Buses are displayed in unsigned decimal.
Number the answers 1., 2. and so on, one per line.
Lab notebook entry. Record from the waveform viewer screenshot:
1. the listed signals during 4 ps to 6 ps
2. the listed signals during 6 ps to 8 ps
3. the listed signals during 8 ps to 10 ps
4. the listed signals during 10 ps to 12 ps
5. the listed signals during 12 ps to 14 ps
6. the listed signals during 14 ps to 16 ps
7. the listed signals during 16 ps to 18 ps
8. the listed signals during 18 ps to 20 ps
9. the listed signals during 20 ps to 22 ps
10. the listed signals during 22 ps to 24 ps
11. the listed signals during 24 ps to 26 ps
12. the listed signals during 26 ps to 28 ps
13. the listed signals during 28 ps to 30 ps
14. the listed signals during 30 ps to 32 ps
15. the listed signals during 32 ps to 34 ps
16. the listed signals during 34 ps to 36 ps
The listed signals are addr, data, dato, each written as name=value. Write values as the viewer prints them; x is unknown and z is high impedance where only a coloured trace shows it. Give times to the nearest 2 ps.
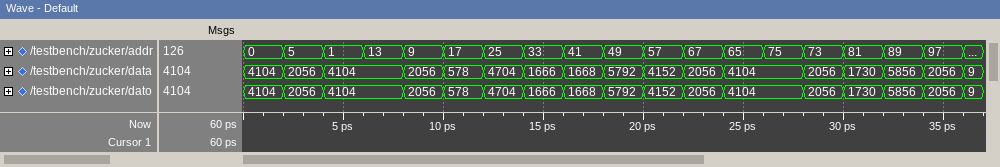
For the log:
1. addr=1, data=4104, dato=4104
2. addr=13, data=4104, dato=4104
3. addr=9, data=2056, dato=2056
4. addr=17, data=578, dato=578
5. addr=25, data=4704, dato=4704
6. addr=33, data=1666, dato=1666
7. addr=41, data=1668, dato=1668
8. addr=49, data=5792, dato=5792
9. addr=57, data=4152, dato=4152
10. addr=67, data=2056, dato=2056
11. addr=65, data=4104, dato=4104
12. addr=75, data=4104, dato=4104
13. addr=73, data=2056, dato=2056
14. addr=81, data=1730, dato=1730
15. addr=89, data=5856, dato=5856
16. addr=97, data=2056, dato=2056
